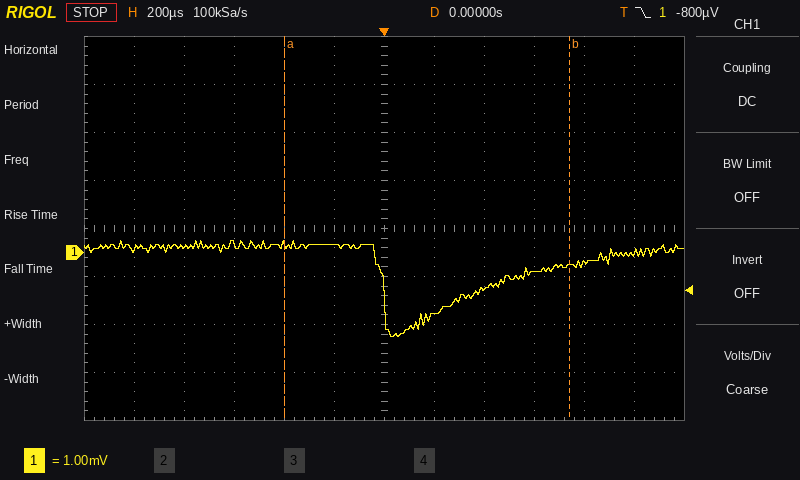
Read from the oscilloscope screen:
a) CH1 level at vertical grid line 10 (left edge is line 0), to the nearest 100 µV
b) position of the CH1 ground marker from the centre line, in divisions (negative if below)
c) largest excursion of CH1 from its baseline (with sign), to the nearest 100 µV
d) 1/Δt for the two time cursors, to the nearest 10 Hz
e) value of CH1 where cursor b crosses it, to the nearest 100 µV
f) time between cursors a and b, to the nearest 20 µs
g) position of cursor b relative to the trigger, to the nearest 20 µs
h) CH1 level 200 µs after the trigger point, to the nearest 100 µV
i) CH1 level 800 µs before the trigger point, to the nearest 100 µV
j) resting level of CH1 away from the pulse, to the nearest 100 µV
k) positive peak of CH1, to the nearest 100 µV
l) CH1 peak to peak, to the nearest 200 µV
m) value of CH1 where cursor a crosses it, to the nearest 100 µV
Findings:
-200 µV
-0.5 div
-1.9 mV
880 Hz
-300 µV
1.14 ms
+740 µs
-1.3 mV
100 µV
100 µV
200 µV
2.0 mV
200 µV
